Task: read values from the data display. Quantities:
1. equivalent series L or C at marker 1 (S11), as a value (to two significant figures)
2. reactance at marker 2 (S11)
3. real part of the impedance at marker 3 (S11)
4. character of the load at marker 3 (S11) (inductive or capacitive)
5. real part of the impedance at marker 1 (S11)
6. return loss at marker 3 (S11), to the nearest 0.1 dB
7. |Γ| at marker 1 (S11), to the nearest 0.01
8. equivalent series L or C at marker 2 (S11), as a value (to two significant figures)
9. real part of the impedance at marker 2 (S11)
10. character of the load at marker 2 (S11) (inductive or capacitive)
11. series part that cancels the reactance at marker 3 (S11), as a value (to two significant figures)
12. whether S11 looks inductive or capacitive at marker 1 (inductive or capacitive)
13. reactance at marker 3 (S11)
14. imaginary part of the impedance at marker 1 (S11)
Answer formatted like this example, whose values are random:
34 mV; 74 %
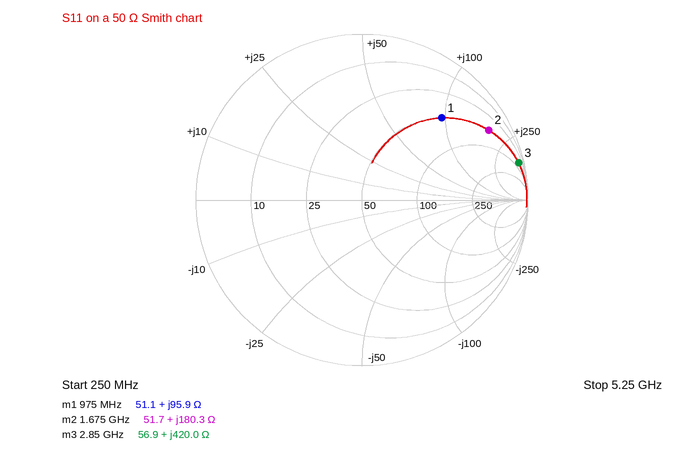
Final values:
16 nH; +180.3 Ω; 56.9 Ω; inductive; 51.1 Ω; 0.3 dB; 0.69; 17 nH; 51.7 Ω; inductive; 130 fF; inductive; +420.0 Ω; +95.9 Ω
